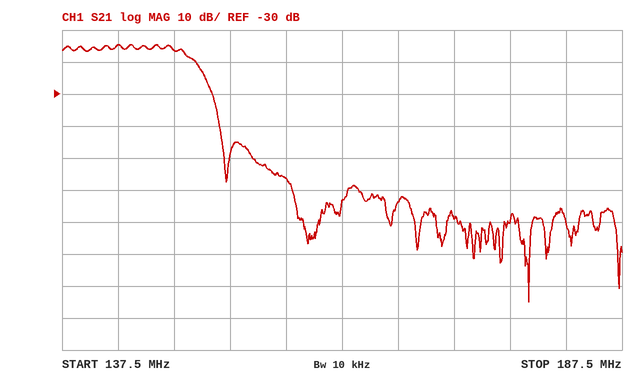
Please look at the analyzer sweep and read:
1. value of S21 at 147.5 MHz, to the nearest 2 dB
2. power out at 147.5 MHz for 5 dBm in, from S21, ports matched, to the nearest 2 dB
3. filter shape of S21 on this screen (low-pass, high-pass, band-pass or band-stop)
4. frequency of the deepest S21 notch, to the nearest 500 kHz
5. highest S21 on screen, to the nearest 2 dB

-16 dB
-12 dBm
low-pass
179.0 MHz
-14 dB
